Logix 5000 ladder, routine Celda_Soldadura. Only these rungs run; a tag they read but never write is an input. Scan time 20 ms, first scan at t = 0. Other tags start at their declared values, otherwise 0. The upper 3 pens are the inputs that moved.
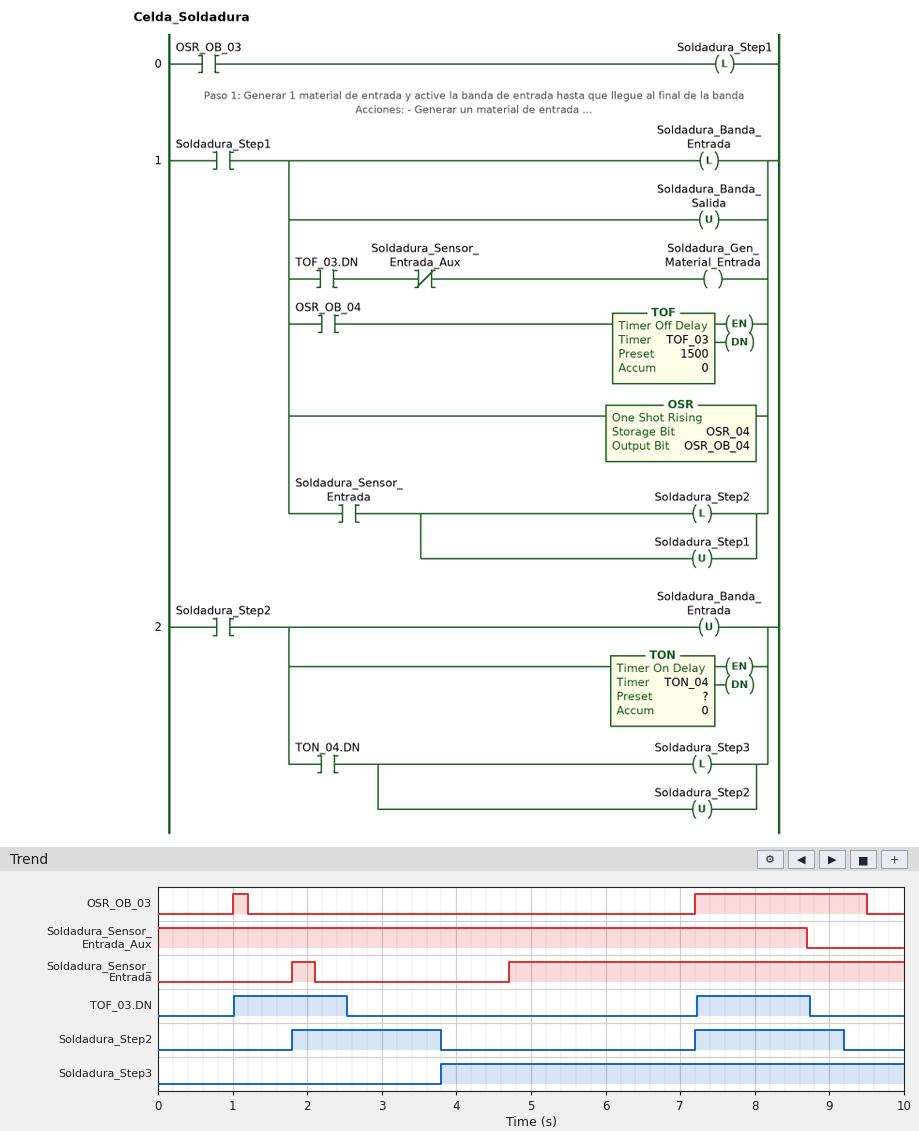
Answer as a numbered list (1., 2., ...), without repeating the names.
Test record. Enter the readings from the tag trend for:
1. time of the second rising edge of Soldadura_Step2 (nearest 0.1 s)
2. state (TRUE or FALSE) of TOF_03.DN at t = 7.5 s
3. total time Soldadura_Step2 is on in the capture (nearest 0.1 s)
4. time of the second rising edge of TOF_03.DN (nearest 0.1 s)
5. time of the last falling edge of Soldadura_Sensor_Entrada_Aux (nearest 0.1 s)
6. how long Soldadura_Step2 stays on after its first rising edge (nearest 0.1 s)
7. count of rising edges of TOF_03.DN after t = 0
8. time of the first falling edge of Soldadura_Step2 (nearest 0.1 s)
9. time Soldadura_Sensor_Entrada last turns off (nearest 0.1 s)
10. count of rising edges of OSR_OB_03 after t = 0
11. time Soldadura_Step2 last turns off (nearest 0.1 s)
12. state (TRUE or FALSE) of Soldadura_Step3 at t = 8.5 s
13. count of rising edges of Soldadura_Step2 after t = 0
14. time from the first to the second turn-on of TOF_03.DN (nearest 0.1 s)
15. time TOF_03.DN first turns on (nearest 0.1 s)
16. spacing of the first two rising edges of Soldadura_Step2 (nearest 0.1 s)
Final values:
1. 7.2 s
2. TRUE
3. 4.0 s
4. 7.2 s
5. 8.7 s
6. 2.0 s
7. 2
8. 3.8 s
9. 2.1 s
10. 2
11. 9.2 s
12. TRUE
13. 2
14. 6.2 s
15. 1.0 s
16. 5.4 s
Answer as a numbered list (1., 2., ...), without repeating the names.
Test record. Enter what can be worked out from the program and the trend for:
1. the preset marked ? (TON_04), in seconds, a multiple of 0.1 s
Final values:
1. 2.0 s
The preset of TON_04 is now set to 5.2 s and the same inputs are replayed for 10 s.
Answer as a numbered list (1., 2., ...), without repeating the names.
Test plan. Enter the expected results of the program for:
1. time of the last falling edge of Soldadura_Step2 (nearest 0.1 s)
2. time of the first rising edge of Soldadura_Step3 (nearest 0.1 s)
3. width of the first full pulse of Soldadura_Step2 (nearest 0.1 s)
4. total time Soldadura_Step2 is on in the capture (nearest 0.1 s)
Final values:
1. 7.0 s
2. 7.0 s
3. 5.2 s
4. 8.0 s
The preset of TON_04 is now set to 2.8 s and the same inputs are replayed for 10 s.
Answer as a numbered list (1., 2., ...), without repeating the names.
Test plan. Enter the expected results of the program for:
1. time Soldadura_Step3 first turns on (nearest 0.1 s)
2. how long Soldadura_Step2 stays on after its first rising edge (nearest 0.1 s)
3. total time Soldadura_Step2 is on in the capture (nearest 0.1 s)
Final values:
1. 4.6 s
2. 2.8 s
3. 5.6 s
